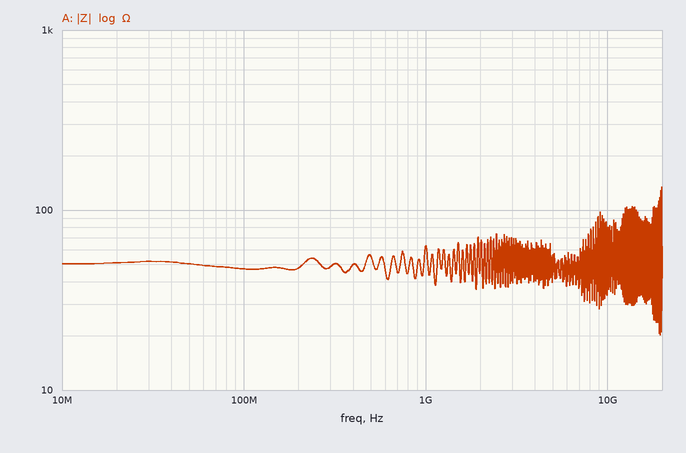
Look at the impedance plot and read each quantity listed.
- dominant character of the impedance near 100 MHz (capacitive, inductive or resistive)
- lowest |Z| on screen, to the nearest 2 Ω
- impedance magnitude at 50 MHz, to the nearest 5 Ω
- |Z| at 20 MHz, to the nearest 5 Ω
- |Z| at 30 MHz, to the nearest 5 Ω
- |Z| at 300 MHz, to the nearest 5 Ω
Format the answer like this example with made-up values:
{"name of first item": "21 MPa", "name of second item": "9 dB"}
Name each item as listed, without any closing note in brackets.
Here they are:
{"dominant character of the impedance near 100 MHz": "resistive", "lowest |Z| on screen, to the nearest 2 Ω": "20 Ω", "impedance magnitude at 50 MHz, to the nearest 5 Ω": "50 Ω", "|Z| at 20 MHz, to the nearest 5 Ω": "50 Ω", "|Z| at 30 MHz, to the nearest 5 Ω": "50 Ω", "|Z| at 300 MHz, to the nearest 5 Ω": "50 Ω"}
